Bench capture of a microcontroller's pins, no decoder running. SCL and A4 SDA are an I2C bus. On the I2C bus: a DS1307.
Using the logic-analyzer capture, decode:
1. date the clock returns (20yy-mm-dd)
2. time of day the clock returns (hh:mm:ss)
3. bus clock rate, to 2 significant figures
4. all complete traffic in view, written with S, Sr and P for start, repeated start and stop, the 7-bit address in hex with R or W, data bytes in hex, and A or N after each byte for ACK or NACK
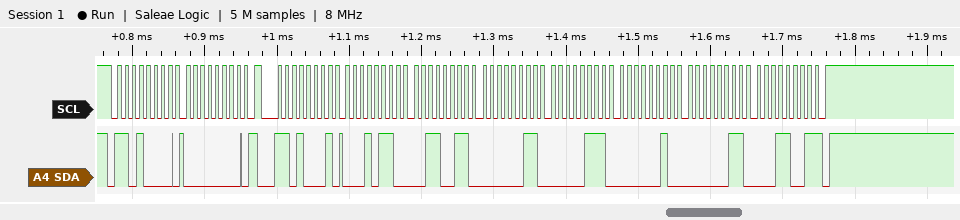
2019-03-02
03:33:16
100 kHz
S 68W A 00 A Sr 68R A 16 A 33 A 03 A 07 A 02 A 03 A 19 N P
